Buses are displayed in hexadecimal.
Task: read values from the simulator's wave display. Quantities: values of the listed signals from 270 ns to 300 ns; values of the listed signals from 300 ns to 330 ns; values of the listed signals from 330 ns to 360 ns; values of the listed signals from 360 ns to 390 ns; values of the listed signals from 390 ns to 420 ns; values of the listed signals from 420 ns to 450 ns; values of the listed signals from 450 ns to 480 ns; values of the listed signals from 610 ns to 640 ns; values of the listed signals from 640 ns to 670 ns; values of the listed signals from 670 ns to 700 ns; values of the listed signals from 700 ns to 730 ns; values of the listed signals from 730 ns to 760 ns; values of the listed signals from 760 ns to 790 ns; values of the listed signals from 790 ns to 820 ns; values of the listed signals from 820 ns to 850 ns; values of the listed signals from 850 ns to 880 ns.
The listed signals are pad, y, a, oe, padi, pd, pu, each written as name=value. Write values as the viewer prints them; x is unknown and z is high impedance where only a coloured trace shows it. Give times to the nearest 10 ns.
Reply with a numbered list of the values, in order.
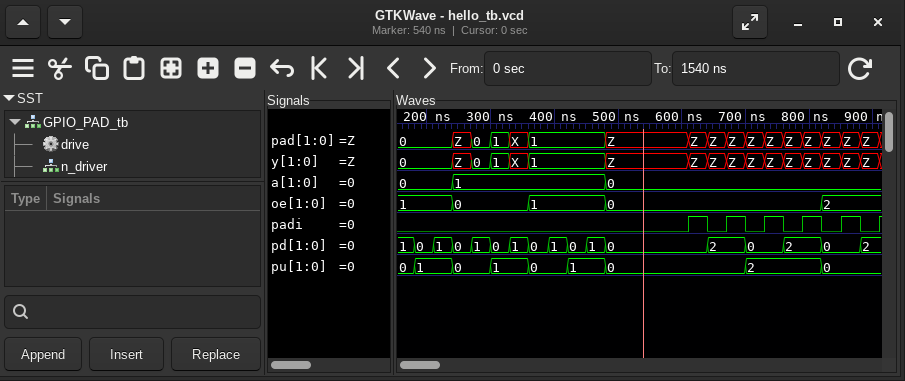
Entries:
1. pad=0, y=0, a=1, oe=0, padi=0, pd=1, pu=0
2. pad=1, y=1, a=1, oe=0, padi=0, pd=0, pu=1
3. pad=X, y=X, a=1, oe=0, padi=0, pd=1, pu=1
4. pad=1, y=1, a=1, oe=1, padi=0, pd=0, pu=0
5. pad=1, y=1, a=1, oe=1, padi=0, pd=1, pu=0
6. pad=1, y=1, a=1, oe=1, padi=0, pd=0, pu=1
7. pad=1, y=1, a=1, oe=1, padi=0, pd=1, pu=1
8. pad=Z, y=Z, a=0, oe=0, padi=1, pd=0, pu=0
9. pad=Z, y=Z, a=0, oe=0, padi=0, pd=2, pu=0
10. pad=Z, y=Z, a=0, oe=0, padi=1, pd=2, pu=0
11. pad=Z, y=Z, a=0, oe=0, padi=0, pd=0, pu=2
12. pad=Z, y=Z, a=0, oe=0, padi=1, pd=0, pu=2
13. pad=Z, y=Z, a=0, oe=0, padi=0, pd=2, pu=2
14. pad=Z, y=Z, a=0, oe=0, padi=1, pd=2, pu=2
15. pad=Z, y=Z, a=0, oe=2, padi=0, pd=0, pu=0
16. pad=Z, y=Z, a=0, oe=2, padi=1, pd=0, pu=0
